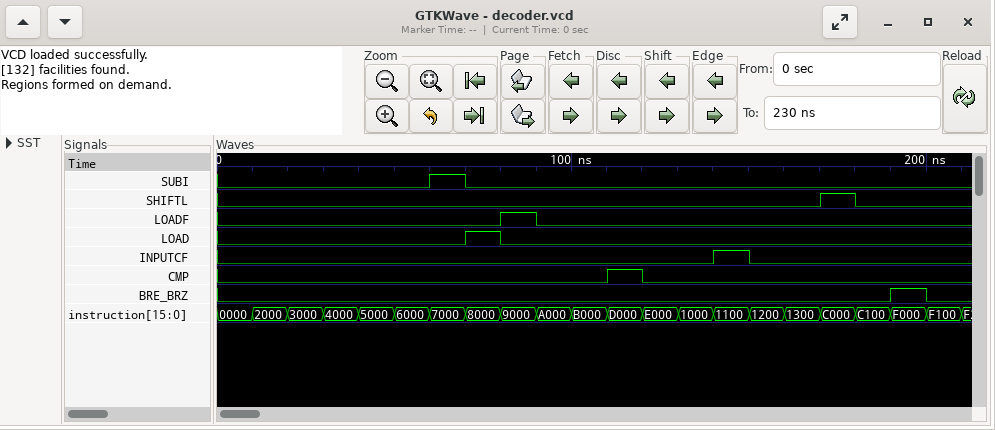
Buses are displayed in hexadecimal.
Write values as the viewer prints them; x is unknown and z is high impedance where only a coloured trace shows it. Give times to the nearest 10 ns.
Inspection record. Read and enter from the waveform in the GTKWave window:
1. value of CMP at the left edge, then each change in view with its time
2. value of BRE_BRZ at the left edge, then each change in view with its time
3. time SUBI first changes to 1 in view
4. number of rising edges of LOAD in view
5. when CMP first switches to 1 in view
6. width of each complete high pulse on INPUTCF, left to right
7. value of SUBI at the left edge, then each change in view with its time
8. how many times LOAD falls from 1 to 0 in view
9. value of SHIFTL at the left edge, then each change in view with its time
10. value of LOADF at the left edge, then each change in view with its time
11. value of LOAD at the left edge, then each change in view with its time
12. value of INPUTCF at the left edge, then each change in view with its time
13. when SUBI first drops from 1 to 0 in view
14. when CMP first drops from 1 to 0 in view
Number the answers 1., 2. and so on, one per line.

1. 0, 1 at 110 ns, 0 at 120 ns
2. 0, 1 at 190 ns, 0 at 200 ns
3. 60 ns
4. 1
5. 110 ns
6. 10 ns
7. 0, 1 at 60 ns, 0 at 70 ns
8. 1
9. 0, 1 at 170 ns, 0 at 180 ns
10. 0, 1 at 80 ns, 0 at 90 ns
11. 0, 1 at 70 ns, 0 at 80 ns
12. 0, 1 at 140 ns, 0 at 150 ns
13. 70 ns
14. 120 ns
